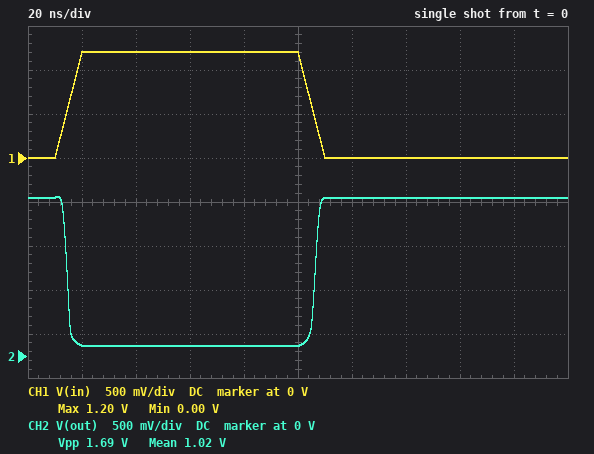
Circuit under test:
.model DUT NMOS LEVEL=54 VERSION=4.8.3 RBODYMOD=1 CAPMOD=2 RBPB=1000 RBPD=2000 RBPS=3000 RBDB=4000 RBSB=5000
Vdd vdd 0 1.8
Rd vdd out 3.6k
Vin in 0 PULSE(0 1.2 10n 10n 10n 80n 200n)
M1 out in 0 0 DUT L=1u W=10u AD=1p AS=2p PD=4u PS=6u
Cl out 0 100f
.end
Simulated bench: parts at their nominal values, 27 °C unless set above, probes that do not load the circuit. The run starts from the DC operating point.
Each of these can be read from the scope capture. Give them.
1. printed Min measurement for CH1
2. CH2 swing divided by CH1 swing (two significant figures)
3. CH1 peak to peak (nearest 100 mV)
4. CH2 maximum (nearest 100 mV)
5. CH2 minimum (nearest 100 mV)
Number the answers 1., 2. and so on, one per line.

1. 0.00 V
2. 1.4
3. 1.2 V
4. 1.8 V
5. 100 mV
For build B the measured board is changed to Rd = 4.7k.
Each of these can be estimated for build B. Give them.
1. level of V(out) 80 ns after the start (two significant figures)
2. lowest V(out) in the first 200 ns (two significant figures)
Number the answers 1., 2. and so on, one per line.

1. 86 mV
2. 85 mV
